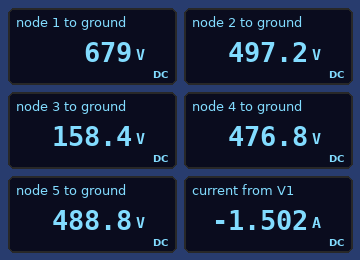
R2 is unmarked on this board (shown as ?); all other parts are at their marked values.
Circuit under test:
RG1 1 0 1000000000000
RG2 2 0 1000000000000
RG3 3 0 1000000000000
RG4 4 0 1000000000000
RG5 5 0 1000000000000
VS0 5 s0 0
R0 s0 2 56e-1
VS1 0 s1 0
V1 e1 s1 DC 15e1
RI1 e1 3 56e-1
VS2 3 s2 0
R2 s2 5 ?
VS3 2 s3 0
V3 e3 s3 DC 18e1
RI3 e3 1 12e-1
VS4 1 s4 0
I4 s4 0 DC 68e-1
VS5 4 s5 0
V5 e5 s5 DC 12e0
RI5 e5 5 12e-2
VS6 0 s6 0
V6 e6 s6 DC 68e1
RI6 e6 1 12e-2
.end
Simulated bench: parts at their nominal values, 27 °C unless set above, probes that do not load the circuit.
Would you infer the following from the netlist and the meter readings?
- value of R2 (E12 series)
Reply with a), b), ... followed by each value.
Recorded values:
a) 220 Ω
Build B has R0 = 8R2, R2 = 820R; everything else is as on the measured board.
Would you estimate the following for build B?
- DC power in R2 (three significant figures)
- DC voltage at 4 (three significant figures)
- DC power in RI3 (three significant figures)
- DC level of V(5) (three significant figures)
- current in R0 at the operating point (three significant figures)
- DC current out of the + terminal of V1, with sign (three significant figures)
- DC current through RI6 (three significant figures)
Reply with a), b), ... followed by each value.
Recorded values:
a) 143 W
b) 483 V
c) 210 mW
d) 495 V
e) 418 mA
f) -418 mA
g) 7.22 A
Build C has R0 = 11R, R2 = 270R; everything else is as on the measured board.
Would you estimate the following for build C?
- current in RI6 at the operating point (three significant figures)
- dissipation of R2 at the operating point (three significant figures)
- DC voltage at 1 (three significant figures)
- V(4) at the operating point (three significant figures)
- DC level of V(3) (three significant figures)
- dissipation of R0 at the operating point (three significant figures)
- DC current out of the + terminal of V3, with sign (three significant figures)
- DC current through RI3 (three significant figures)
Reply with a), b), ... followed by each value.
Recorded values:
a) 8.01 A
b) 397 W
c) 679 V
d) 472 V
e) 157 V
f) 16.2 W
g) -1.21 A
h) 1.21 A
